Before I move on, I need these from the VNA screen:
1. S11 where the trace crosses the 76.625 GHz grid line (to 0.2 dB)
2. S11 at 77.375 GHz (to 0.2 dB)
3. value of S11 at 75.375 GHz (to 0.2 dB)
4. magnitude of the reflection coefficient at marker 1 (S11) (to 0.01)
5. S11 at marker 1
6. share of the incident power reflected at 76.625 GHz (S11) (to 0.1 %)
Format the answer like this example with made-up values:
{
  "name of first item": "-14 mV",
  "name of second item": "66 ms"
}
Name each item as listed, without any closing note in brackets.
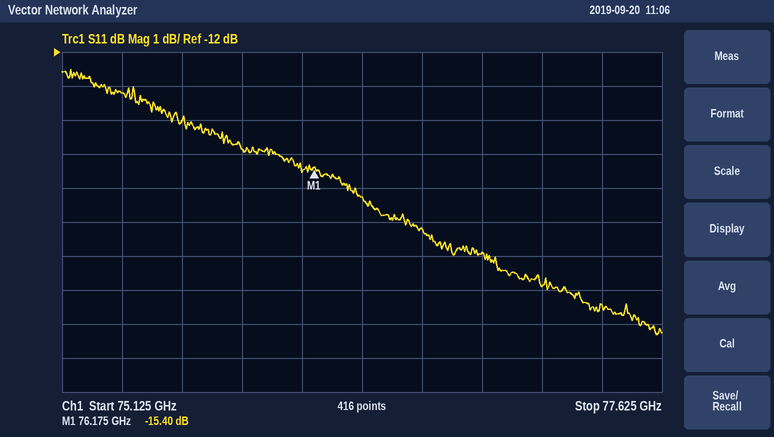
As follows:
{
  "S11 where the trace crosses the 76.625 GHz grid line": "-17.2 dB",
  "S11 at 77.375 GHz": "-19.4 dB",
  "value of S11 at 75.375 GHz": "-13.2 dB",
  "magnitude of the reflection coefficient at marker 1 (S11)": "0.17",
  "S11 at marker 1": "-15.40 dB",
  "share of the incident power reflected at 76.625 GHz (S11)": "1.9 %"
}
